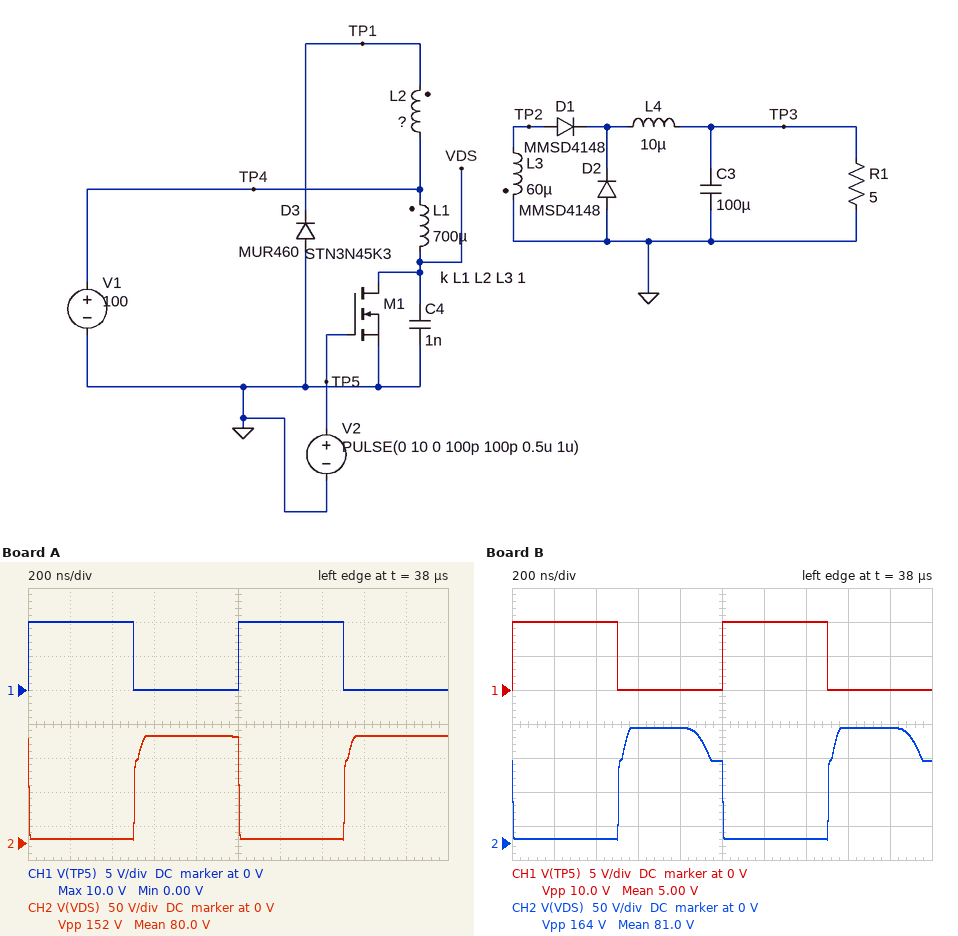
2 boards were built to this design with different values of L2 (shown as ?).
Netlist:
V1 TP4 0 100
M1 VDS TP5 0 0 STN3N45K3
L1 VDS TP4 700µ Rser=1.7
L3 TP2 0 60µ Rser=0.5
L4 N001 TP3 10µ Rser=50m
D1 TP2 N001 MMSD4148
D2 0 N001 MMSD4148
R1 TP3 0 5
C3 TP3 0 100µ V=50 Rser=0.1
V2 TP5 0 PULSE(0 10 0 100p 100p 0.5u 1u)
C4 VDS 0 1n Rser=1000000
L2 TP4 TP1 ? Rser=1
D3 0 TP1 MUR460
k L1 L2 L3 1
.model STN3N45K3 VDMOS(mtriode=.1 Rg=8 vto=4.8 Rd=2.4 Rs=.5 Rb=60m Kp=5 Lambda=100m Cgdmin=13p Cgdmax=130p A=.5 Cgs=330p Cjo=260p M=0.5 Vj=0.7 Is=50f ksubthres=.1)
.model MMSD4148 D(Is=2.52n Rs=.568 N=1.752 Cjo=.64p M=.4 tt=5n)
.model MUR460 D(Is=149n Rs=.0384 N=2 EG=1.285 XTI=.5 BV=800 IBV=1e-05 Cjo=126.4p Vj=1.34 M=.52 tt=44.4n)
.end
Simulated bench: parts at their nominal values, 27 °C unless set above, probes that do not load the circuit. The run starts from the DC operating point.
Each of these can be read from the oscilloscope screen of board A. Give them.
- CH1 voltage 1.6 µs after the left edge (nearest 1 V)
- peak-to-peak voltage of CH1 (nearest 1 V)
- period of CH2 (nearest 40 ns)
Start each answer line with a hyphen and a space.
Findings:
- 0 V
- 10 V
- 1.00 µs
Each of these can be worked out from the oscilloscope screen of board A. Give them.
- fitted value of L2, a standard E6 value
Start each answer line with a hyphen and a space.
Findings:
- 2.2 mH
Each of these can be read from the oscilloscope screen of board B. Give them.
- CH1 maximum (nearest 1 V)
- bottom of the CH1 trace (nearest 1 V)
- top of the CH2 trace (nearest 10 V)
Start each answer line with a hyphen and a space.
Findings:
- 10 V
- 0 V
- 170 V
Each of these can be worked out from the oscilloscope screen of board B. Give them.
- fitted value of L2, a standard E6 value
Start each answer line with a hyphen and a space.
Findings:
- 1.5 mH
